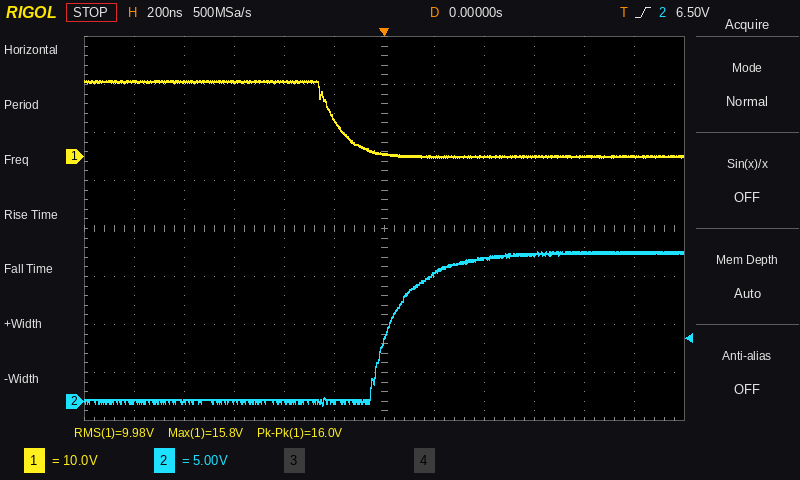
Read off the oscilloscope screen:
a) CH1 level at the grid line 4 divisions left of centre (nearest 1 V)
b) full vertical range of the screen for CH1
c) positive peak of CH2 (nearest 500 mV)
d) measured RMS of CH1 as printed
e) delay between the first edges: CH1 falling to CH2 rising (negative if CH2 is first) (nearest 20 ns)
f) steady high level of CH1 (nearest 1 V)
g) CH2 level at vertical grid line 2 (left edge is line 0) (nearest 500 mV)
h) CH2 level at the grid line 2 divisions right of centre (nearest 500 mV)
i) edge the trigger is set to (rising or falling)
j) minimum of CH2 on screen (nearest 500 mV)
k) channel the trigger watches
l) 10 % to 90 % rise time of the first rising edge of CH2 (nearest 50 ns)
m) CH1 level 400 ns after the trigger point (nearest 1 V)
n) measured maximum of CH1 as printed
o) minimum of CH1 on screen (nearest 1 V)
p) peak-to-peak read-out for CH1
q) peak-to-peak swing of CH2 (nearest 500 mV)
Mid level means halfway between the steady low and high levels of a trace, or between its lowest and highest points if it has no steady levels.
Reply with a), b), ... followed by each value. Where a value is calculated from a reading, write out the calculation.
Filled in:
a) 16 V
b) 80 V
c) 15.5 V
d) 9.98 V
e) +220 ns
f) 16 V
g) 0.0 V
h) 15.0 V
i) rising
j) -500 mV
k) CH2
l) 300 ns
m) 0 V
n) 15.8 V
o) 0 V
p) 16.0 V
q) 15.5 V − (-500 mV) = 16.0 V
